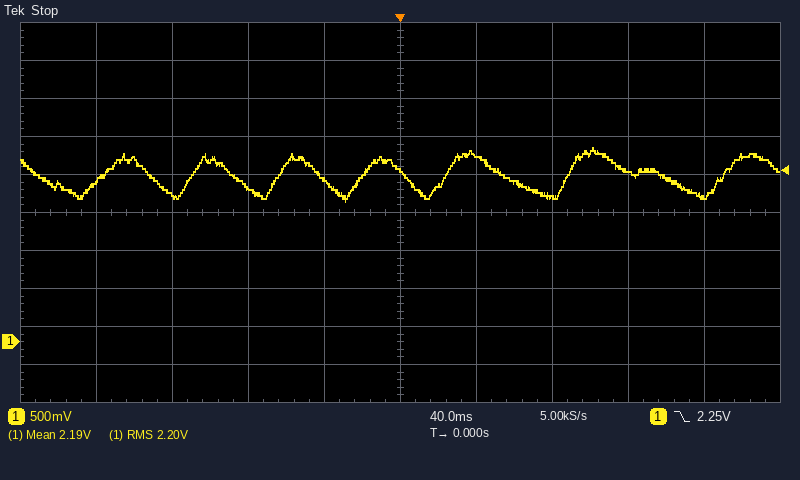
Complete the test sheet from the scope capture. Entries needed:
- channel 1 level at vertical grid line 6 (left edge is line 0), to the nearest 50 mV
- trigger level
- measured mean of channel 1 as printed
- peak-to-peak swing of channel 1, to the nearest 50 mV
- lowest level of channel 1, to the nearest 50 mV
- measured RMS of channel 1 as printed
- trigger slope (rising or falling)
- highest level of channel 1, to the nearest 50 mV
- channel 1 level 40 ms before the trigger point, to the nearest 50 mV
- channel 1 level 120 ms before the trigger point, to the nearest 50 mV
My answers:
2.45 V
2.25 V
2.19 V
700 mV
1.85 V
2.20 V
falling
2.55 V
2.10 V
1.90 V
